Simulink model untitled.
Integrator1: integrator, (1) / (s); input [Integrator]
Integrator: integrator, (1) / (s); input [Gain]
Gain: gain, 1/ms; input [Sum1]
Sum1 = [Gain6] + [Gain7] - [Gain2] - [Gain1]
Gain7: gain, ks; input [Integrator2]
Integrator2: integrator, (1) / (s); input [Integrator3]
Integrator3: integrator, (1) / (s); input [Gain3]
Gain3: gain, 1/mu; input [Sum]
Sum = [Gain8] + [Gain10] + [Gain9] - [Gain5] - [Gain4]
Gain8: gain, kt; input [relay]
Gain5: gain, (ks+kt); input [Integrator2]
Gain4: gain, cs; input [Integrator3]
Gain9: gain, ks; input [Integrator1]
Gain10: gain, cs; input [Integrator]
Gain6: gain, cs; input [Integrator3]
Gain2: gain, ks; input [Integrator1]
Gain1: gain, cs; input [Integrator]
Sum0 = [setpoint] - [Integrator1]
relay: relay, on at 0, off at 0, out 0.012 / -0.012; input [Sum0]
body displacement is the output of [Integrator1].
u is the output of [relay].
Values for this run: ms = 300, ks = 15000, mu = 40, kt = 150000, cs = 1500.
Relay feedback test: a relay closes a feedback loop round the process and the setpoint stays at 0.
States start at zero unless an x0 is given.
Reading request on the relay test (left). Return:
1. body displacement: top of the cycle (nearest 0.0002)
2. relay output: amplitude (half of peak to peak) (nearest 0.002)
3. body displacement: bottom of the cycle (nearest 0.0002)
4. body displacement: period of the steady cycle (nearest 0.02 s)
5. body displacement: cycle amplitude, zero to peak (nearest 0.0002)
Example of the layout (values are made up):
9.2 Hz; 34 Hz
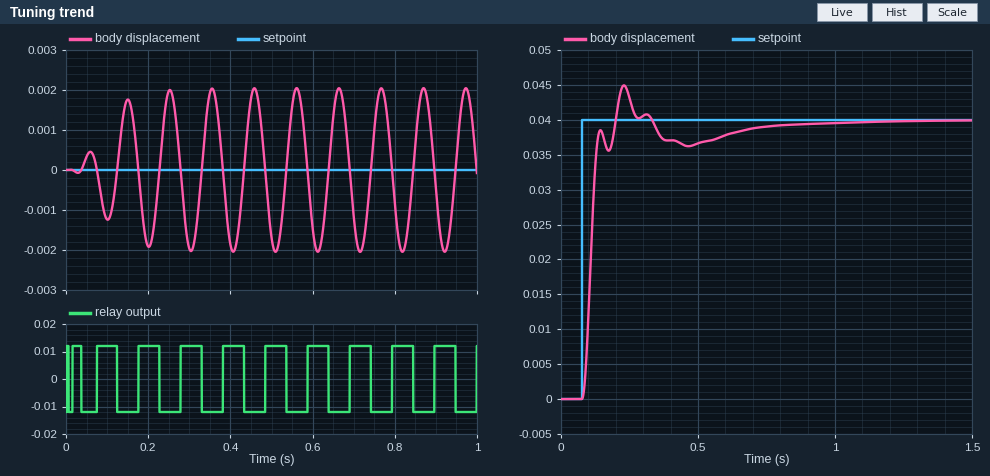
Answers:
0.0020; 0.012; -0.0020; 0.10 s; 0.0020
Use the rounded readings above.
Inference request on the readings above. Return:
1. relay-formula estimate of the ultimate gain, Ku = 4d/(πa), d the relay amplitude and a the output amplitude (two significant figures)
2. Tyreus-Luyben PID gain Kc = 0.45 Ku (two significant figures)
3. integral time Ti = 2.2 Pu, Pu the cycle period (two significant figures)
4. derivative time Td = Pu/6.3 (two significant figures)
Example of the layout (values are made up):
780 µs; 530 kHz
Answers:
7.6; 3.4; 0.22 s; 0.016 s
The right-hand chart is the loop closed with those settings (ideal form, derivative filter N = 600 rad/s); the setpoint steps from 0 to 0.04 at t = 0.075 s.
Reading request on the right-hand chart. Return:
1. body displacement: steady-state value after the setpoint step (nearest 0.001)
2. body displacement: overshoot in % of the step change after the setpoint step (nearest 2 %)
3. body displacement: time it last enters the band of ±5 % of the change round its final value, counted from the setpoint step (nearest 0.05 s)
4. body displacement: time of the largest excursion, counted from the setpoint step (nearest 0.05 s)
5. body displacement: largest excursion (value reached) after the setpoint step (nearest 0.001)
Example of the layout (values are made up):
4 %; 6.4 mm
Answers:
0.040; 12 %; 0.55 s; 0.15 s; 0.045
